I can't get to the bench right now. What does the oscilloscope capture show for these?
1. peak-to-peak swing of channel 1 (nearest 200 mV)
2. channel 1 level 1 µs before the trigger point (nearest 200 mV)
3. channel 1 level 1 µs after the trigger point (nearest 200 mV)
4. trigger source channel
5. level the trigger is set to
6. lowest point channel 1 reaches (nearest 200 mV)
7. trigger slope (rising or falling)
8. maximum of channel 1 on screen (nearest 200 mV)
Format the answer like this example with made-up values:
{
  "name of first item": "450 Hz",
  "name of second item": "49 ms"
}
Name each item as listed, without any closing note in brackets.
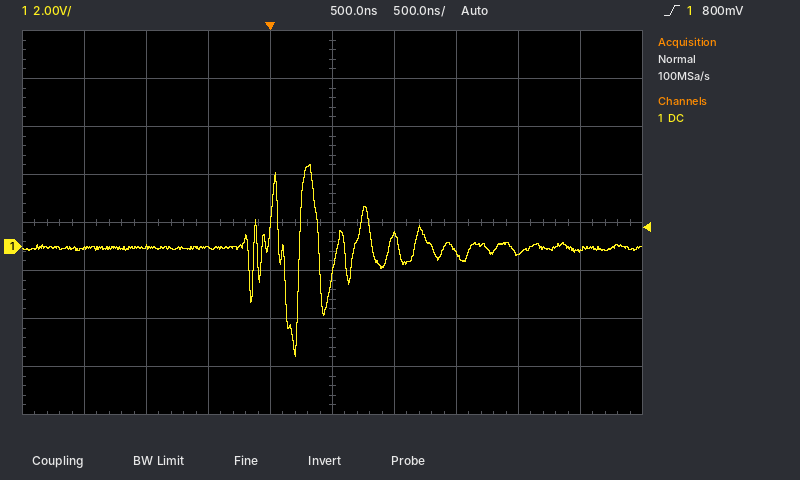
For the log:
{
  "peak-to-peak swing of channel 1": "8.0 V",
  "channel 1 level 1 µs before the trigger point": "0.0 V",
  "channel 1 level 1 µs after the trigger point": "400 mV",
  "trigger source channel": "channel 1",
  "level the trigger is set to": "800 mV",
  "lowest point channel 1 reaches": "-4.6 V",
  "trigger slope": "rising",
  "maximum of channel 1 on screen": "3.4 V"
}
